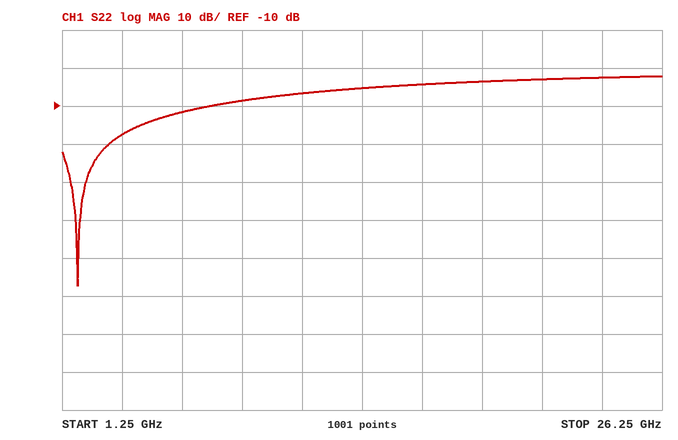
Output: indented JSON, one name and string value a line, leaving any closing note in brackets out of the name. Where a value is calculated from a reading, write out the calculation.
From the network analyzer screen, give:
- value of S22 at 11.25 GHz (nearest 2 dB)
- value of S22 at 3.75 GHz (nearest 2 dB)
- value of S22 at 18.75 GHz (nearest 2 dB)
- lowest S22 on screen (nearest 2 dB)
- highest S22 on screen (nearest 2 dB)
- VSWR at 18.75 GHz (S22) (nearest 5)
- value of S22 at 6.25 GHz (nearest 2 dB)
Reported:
{
  "value of S22 at 11.25 GHz": "-6 dB",
  "value of S22 at 3.75 GHz": "-18 dB",
  "value of S22 at 18.75 GHz": "-4 dB",
  "lowest S22 on screen": "-58 dB",
  "highest S22 on screen": "-2 dB",
  "VSWR at 18.75 GHz (S22)": "|Γ| = 10^(-4/20) = 0.6310; VSWR = (1 + 0.6310)/(1 − 0.6310) ≈ 4.42, so 5 to the nearest 5",
  "value of S22 at 6.25 GHz": "-12 dB"
}
